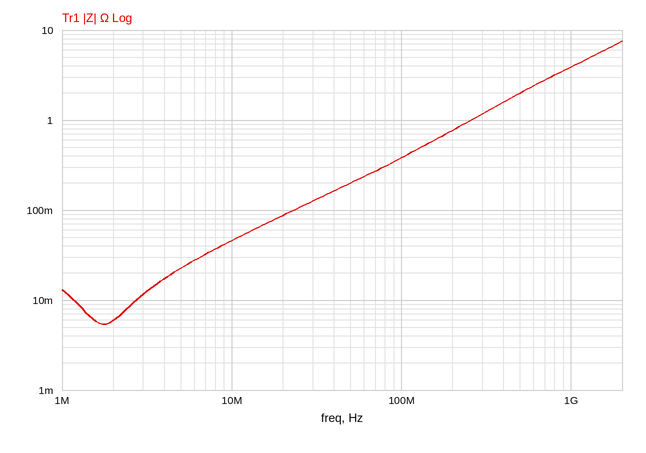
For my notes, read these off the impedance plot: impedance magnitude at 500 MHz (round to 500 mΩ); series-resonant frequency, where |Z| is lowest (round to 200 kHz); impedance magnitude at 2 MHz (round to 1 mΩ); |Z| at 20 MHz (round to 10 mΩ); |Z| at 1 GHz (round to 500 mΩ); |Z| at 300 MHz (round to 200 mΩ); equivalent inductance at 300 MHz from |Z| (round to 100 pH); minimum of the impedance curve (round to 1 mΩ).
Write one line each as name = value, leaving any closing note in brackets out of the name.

impedance magnitude at 500 MHz = 2.0 Ω
series-resonant frequency, where |Z| is lowest = 1.8 MHz
impedance magnitude at 2 MHz = 6 mΩ
|Z| at 20 MHz = 90 mΩ
|Z| at 1 GHz = 4.0 Ω
|Z| at 300 MHz = 1.2 Ω
equivalent inductance at 300 MHz from |Z| = 600 pH
minimum of the impedance curve = 5 mΩ
